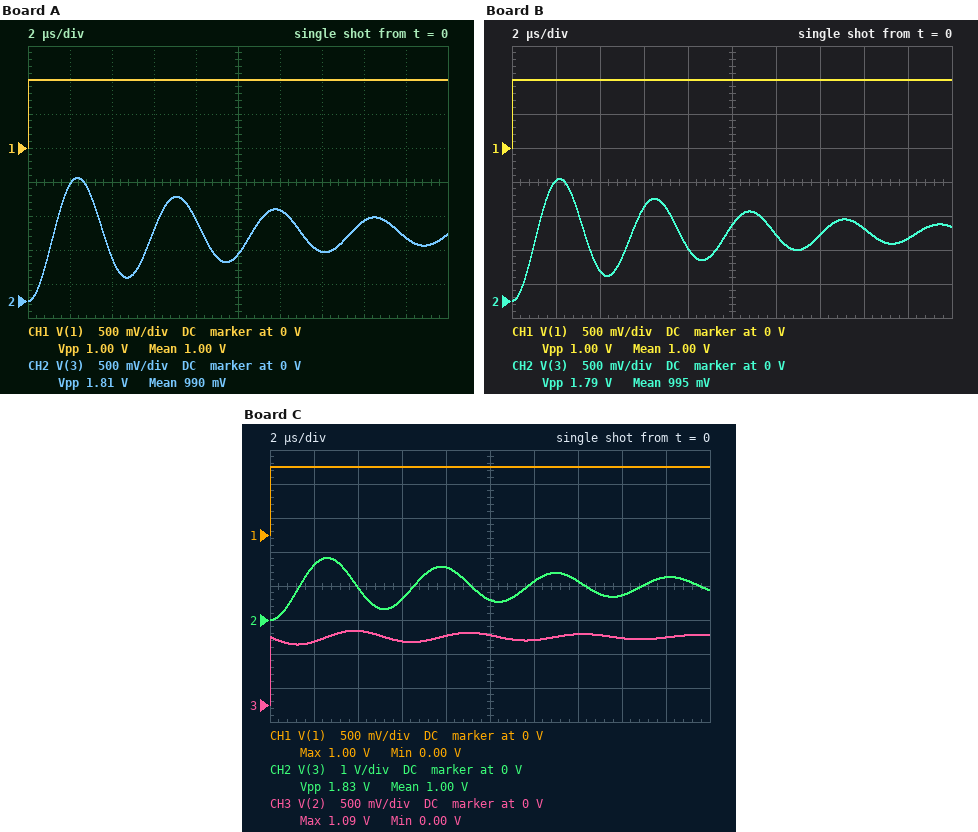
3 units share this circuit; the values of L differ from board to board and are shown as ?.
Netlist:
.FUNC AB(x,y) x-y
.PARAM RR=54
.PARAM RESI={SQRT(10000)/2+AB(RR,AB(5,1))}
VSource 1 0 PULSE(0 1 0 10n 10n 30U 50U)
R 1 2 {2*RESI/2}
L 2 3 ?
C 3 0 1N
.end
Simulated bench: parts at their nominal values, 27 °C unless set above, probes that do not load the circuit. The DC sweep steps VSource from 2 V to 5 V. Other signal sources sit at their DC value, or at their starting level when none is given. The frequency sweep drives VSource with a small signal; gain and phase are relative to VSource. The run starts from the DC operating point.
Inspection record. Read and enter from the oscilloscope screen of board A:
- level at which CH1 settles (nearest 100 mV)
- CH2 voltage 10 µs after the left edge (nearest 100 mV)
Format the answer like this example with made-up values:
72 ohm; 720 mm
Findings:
1.0 V; 700 mV
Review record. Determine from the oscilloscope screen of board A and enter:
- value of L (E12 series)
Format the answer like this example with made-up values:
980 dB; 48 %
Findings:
560 µH
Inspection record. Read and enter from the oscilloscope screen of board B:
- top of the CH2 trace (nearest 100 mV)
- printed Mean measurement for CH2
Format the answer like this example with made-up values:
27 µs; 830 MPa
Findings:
1.8 V; 995 mV
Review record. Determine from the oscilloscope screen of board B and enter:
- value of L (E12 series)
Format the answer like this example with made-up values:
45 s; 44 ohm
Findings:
470 µH
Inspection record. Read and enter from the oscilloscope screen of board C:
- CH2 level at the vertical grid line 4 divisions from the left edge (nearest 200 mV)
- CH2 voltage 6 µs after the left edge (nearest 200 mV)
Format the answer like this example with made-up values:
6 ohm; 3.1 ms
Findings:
1.6 V; 600 mV
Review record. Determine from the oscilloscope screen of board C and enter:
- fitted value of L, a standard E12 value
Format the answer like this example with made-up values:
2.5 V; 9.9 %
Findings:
680 µH
